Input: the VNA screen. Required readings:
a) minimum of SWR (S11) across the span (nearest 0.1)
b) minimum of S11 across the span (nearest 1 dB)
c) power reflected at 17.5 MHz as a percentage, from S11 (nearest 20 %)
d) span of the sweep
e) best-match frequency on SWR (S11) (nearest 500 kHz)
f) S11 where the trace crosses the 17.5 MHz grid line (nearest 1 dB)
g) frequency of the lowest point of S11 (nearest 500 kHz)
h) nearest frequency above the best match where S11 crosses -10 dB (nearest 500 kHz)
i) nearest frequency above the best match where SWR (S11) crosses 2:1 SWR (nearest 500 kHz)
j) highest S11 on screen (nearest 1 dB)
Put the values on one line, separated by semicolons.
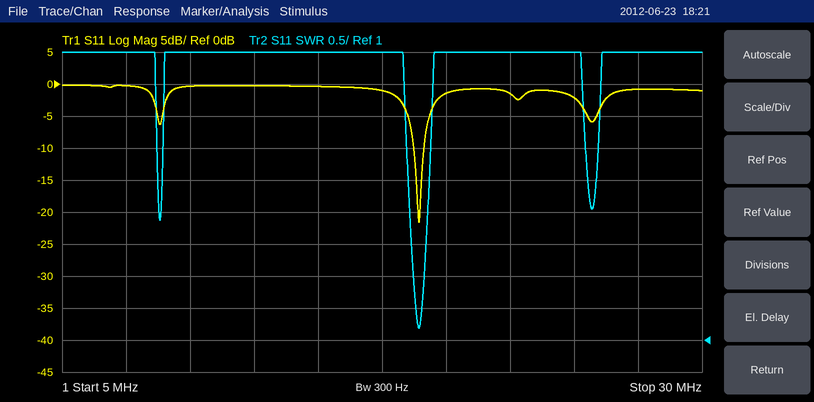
1.2; -22 dB; 80 %; 25 MHz; 19.0 MHz; -1 dB; 19.0 MHz; 19.0 MHz; 19.0 MHz; 0 dB
